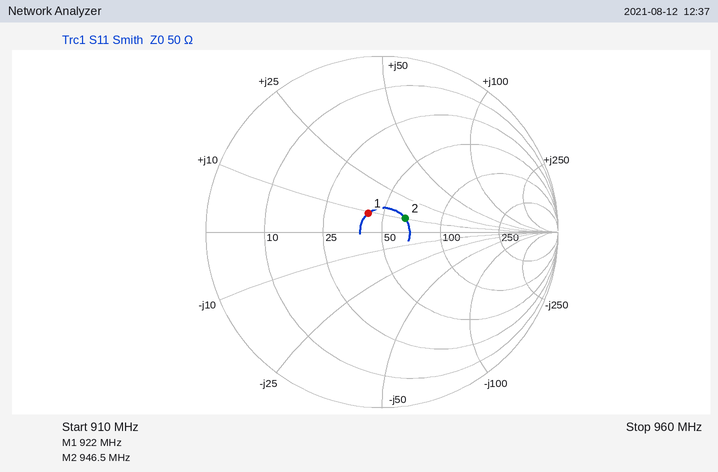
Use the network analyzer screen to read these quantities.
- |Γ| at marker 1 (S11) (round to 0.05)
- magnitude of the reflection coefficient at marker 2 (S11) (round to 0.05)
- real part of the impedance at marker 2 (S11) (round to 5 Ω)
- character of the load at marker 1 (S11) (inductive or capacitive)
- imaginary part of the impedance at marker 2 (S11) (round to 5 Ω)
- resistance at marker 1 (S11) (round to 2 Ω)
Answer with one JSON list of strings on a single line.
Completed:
["0.15", "0.15", "65 Ω", "inductive", "+10 Ω", "42 Ω"]
